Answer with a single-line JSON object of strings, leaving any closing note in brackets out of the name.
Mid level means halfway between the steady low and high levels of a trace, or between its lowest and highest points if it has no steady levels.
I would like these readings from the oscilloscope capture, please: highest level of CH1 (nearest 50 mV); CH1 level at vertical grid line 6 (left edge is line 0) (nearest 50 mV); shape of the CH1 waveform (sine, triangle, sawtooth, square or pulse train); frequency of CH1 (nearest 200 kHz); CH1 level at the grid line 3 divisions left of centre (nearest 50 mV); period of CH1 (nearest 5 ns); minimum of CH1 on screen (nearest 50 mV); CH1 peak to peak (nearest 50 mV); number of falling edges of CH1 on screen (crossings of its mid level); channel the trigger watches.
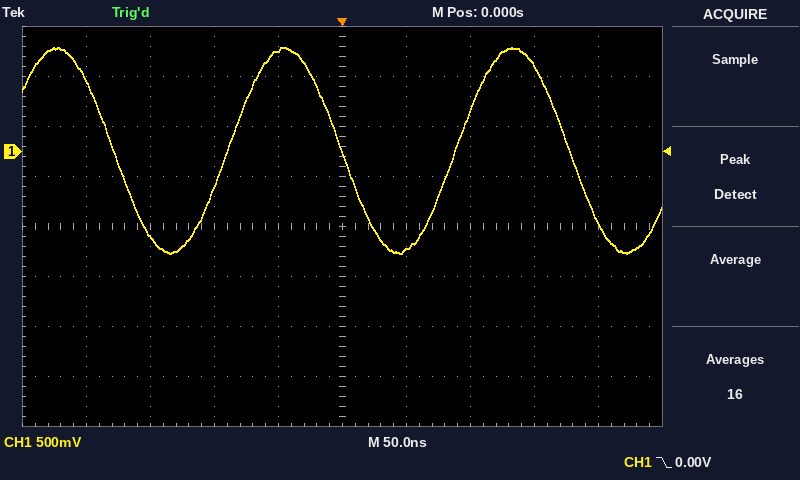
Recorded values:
{"highest level of CH1": "1.05 V", "CH1 level at vertical grid line 6 (left edge is line 0)": "-1.00 V", "shape of the CH1 waveform": "sine", "frequency of CH1": "5.6 MHz", "CH1 level at the grid line 3 divisions left of centre": "-850 mV", "period of CH1": "180 ns", "minimum of CH1 on screen": "-1.00 V", "CH1 peak to peak": "2.05 V", "number of falling edges of CH1 on screen": "3", "channel the trigger watches": "CH1"}
